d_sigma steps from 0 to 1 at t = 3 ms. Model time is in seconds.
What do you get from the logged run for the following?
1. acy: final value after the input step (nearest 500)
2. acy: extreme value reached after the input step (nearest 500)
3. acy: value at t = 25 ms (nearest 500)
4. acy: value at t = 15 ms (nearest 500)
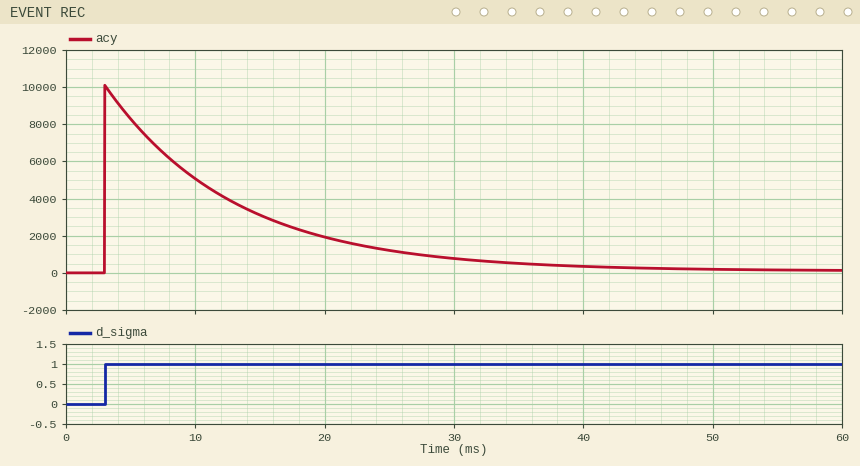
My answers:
0
10000
1000
3000
